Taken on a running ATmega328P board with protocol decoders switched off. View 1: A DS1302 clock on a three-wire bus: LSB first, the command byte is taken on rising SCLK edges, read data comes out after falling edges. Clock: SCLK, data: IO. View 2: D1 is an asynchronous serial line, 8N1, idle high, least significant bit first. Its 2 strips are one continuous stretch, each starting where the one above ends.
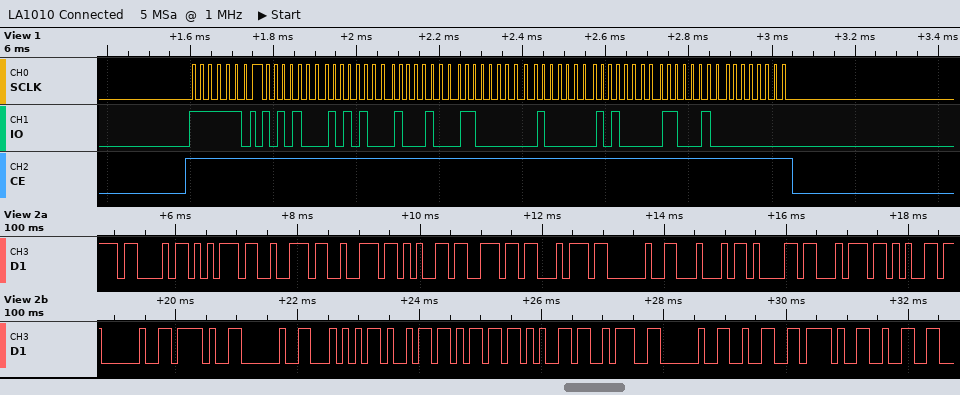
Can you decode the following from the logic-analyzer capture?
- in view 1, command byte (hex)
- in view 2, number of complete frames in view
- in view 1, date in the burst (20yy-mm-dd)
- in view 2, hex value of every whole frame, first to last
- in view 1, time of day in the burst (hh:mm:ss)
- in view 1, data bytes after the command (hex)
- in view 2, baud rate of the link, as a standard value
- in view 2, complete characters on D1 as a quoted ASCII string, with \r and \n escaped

0xBF
24
2023-02-03
0x43 0x75 0x72 0x72 0x65 0x6E 0x74 0x20 0x44 0x61 0x74 0x65 0x20 0x2F 0x20 0x54 0x69 0x6D 0x65 0x3A 0x20 0x32 0x2F 0x32
11:15:15
15 15 11 03 02 05 23 00
9600 baud
"Current Date / Time: 2/2"
